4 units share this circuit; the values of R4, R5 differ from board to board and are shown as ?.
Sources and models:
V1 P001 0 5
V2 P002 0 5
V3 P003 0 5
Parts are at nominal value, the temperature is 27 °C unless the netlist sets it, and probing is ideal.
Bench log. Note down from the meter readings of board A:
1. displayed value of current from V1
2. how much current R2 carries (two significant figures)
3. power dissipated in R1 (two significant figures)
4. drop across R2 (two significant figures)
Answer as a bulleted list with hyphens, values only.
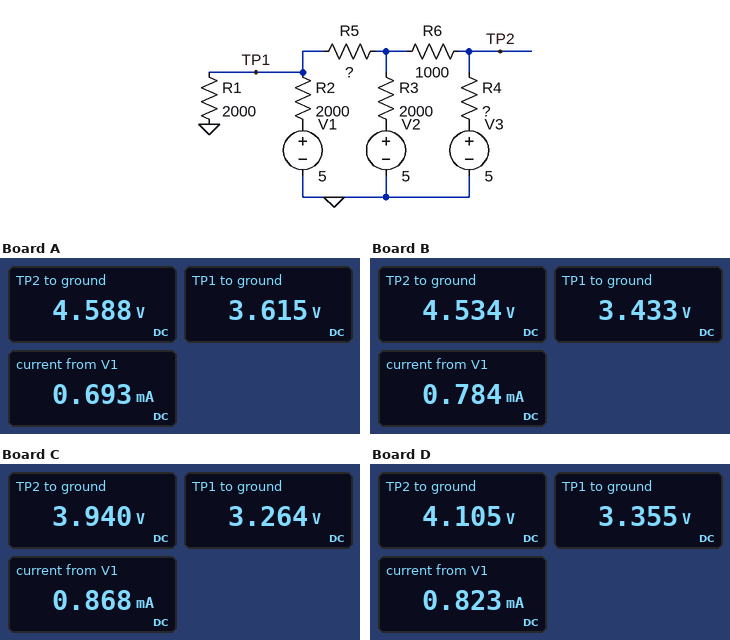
- 0.693 mA
- 690 µA
- 6.5 mW
- 1.4 V
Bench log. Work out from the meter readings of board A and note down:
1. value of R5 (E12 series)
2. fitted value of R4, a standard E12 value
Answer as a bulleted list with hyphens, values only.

- 330 Ω
- 680 Ω
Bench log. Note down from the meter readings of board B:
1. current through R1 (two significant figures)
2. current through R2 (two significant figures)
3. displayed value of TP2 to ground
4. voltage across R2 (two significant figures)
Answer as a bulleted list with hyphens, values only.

- 1.7 mA
- 780 µA
- 4.534 V
- 1.6 V
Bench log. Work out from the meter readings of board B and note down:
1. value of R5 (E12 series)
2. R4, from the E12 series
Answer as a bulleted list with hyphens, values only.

- 680 Ω
- 1 kΩ
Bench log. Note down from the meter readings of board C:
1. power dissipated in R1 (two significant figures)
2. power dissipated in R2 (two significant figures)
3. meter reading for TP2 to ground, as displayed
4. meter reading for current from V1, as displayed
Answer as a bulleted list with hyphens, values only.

- 5.3 mW
- 1.5 mW
- 3.940 V
- 0.868 mA
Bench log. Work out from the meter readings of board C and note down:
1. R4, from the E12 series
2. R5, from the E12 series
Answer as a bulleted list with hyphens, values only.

- 6.8 kΩ
- 680 Ω
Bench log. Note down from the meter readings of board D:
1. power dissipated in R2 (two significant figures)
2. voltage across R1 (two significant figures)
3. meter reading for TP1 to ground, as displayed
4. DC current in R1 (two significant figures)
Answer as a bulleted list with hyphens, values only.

- 1.4 mW
- 3.4 V
- 3.355 V
- 1.7 mA
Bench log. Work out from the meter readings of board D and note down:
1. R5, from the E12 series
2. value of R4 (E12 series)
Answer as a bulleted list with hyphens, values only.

- 560 Ω
- 3.3 kΩ
